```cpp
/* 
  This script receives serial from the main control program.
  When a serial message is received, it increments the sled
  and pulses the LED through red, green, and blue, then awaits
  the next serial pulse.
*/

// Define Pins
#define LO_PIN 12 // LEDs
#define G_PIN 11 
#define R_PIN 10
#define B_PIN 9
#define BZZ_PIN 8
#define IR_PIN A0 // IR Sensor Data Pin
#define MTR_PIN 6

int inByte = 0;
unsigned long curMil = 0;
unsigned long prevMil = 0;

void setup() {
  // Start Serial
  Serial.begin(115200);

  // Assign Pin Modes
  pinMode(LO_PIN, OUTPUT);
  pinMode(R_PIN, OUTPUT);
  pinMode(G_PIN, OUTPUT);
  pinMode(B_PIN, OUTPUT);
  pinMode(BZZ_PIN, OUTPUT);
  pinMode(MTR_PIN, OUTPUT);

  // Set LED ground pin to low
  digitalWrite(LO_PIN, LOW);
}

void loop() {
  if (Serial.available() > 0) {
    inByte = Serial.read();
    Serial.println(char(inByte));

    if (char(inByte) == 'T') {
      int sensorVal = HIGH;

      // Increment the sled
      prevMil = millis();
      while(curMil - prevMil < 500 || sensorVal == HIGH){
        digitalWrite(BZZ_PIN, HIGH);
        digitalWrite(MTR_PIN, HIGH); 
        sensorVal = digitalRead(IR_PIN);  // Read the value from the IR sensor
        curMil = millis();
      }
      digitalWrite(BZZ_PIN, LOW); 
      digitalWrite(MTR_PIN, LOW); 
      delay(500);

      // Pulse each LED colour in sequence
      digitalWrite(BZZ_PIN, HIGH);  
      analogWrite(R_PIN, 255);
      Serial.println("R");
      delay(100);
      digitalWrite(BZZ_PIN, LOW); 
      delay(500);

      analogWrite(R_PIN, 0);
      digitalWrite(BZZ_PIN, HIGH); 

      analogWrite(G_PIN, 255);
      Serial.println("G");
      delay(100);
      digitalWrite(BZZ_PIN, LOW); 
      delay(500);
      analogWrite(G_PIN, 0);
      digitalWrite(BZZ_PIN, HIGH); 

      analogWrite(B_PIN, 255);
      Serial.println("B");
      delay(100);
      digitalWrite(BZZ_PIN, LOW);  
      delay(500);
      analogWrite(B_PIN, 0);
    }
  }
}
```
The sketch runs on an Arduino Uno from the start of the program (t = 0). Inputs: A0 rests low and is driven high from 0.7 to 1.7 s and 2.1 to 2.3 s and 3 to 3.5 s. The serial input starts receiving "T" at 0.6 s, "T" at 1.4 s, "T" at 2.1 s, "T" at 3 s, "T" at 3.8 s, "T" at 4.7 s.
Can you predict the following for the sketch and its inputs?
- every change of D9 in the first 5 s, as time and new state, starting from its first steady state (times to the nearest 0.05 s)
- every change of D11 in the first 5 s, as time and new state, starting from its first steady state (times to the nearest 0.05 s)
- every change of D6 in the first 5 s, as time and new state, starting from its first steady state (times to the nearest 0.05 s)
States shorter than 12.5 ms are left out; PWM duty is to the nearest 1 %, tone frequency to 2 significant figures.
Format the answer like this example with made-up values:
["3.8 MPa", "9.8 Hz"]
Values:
["0 s low; 3.4 s high; 4 s low", "0 s low; 2.8 s high; 3.4 s low", "0 s low; 0.6 s high; 1.7 s low; 4 s high; 4.5 s low"]
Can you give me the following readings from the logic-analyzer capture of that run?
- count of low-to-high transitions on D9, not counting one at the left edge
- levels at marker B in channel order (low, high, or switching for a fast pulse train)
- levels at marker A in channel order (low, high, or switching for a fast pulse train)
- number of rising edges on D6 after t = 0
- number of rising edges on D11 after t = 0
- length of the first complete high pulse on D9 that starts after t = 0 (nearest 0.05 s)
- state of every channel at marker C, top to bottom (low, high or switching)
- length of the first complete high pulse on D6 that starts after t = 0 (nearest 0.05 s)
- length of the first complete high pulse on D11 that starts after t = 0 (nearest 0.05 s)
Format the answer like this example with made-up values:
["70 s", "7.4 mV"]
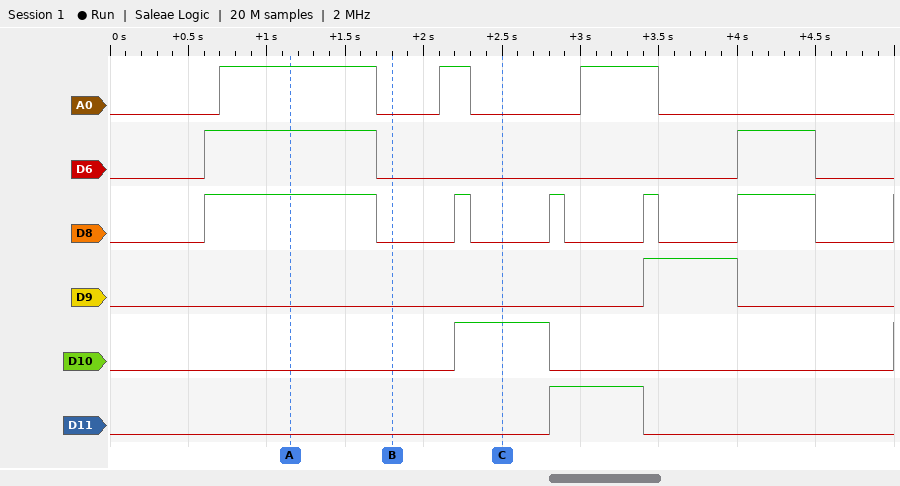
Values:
["1", "A0 low, D6 low, D8 low, D9 low, D10 low, D11 low", "A0 high, D6 high, D8 high, D9 low, D10 low, D11 low", "2", "1", "0.60 s", "A0 low, D6 low, D8 low, D9 low, D10 high, D11 low", "1.10 s", "0.60 s"]
